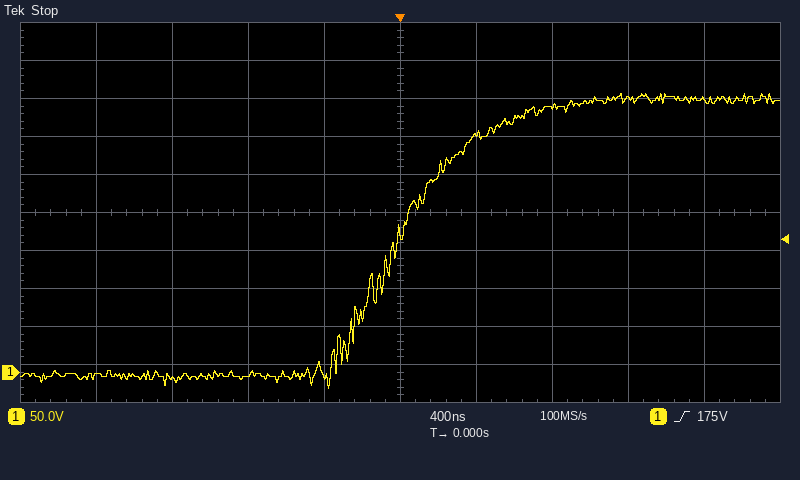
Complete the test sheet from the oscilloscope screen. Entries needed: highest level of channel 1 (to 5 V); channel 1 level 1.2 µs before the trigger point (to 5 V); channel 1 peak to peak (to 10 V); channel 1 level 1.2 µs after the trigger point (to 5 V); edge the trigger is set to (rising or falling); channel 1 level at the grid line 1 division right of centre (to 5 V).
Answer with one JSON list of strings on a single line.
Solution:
["365 V", "-10 V", "390 V", "360 V", "rising", "315 V"]
